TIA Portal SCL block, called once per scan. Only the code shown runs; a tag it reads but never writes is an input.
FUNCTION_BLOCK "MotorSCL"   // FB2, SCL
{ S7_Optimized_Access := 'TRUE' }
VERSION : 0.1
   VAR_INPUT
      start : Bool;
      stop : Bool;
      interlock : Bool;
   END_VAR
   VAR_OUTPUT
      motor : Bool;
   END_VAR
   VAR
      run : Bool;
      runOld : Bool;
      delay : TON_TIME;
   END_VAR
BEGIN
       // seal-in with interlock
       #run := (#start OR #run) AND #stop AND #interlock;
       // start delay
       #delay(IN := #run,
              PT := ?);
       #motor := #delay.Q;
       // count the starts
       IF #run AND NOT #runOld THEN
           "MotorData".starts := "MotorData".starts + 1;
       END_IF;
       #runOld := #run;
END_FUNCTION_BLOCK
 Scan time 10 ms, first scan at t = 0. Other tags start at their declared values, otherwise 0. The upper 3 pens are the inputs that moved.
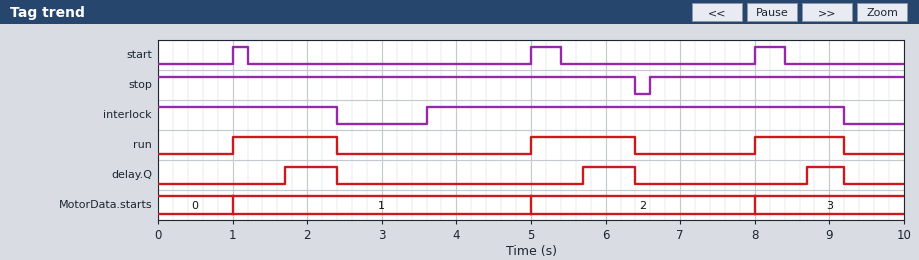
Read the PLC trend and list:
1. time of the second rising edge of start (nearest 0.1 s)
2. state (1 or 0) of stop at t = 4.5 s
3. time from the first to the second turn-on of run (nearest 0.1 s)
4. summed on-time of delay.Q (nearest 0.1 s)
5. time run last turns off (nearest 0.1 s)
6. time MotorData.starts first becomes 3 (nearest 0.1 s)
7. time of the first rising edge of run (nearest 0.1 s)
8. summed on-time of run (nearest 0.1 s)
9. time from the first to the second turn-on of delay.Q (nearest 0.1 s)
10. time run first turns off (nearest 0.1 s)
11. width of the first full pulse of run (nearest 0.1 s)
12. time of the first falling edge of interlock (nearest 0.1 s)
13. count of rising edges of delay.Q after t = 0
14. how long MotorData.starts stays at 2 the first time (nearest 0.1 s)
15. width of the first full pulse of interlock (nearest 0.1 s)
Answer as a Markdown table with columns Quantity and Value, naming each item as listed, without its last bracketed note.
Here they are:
| Quantity | Value |
|---|---|
| time of the second rising edge of start | 5.0 s |
| state (1 or 0) of stop at t = 4.5 s | 1 |
| time from the first to the second turn-on of run | 4.0 s |
| summed on-time of delay.Q | 1.9 s |
| time run last turns off | 9.2 s |
| time MotorData.starts first becomes 3 | 8.0 s |
| time of the first rising edge of run | 1.0 s |
| summed on-time of run | 4.0 s |
| time from the first to the second turn-on of delay.Q | 4.0 s |
| time run first turns off | 2.4 s |
| width of the first full pulse of run | 1.4 s |
| time of the first falling edge of interlock | 2.4 s |
| count of rising edges of delay.Q after t = 0 | 3 |
| how long MotorData.starts stays at 2 the first time | 3.0 s |
| width of the first full pulse of interlock | 5.6 s |
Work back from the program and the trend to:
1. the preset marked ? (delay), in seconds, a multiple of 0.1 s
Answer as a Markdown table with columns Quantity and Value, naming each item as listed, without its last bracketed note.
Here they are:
| Quantity | Value |
|---|---|
| the preset marked ? (delay), in seconds, a multiple of 0.1 s | 0.7 s |
